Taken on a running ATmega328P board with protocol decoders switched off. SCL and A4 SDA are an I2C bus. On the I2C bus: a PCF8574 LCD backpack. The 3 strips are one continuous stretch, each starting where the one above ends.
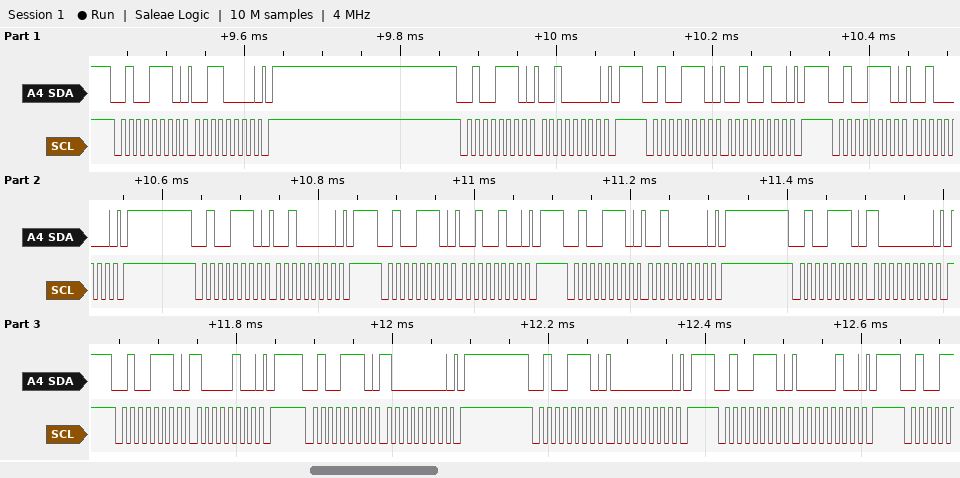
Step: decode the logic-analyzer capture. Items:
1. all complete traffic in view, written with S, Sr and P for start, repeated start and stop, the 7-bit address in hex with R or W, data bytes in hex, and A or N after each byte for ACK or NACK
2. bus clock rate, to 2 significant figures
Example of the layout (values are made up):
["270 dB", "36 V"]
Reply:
["S 27W A 30 A P S 27W A 20 A P S 27W A 24 A P S 27W A 20 A P S 27W A 20 A P S 27W A 24 A P S 27W A 20 A P S 27W A 80 A P S 27W A 84 A P S 27W A 80 A P S 27W A 00 A P S 27W A 04 A P", "100 kHz"]
